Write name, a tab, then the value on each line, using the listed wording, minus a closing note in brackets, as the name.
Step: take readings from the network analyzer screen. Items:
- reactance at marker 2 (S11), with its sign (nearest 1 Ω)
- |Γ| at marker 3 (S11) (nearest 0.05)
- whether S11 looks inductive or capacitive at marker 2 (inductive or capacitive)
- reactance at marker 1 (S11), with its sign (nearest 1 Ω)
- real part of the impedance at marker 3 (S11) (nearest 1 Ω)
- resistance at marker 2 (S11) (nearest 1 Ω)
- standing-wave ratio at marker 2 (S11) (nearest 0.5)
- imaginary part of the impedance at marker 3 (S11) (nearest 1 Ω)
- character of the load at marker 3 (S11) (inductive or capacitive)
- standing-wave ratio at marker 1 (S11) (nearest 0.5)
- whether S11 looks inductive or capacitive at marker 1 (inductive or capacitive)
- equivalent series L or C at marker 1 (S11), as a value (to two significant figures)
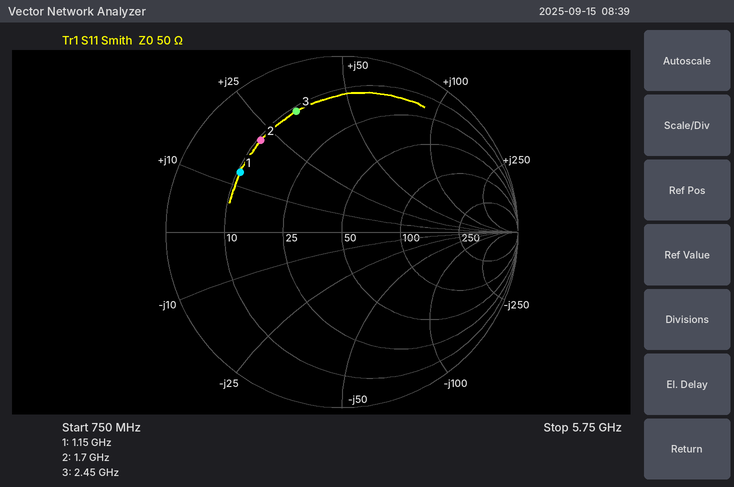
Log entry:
reactance at marker 2 (S11), with its sign	+22 Ω
|Γ| at marker 3 (S11)	0.75
whether S11 looks inductive or capacitive at marker 2	inductive
reactance at marker 1 (S11), with its sign	+13 Ω
real part of the impedance at marker 3 (S11)	11 Ω
resistance at marker 2 (S11)	11 Ω
standing-wave ratio at marker 2 (S11)	5.5
imaginary part of the impedance at marker 3 (S11)	+33 Ω
character of the load at marker 3 (S11)	inductive
standing-wave ratio at marker 1 (S11)	5.0
whether S11 looks inductive or capacitive at marker 1	inductive
equivalent series L or C at marker 1 (S11), as a value	1.8 nH
